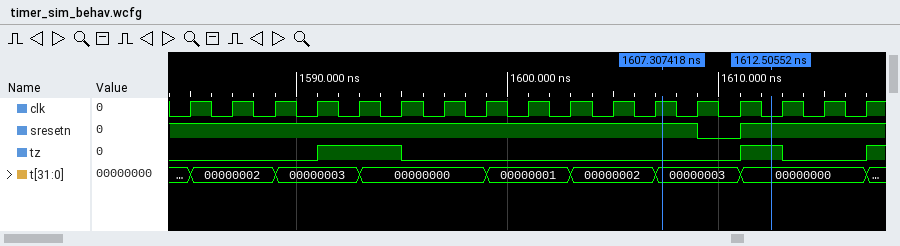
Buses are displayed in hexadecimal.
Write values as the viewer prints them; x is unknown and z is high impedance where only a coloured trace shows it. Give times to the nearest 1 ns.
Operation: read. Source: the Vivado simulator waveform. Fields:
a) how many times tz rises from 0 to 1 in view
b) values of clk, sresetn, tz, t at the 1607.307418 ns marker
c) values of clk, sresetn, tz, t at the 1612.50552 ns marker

3
clk=1, sresetn=1, tz=0, t=00000003
clk=0, sresetn=1, tz=1, t=00000000
